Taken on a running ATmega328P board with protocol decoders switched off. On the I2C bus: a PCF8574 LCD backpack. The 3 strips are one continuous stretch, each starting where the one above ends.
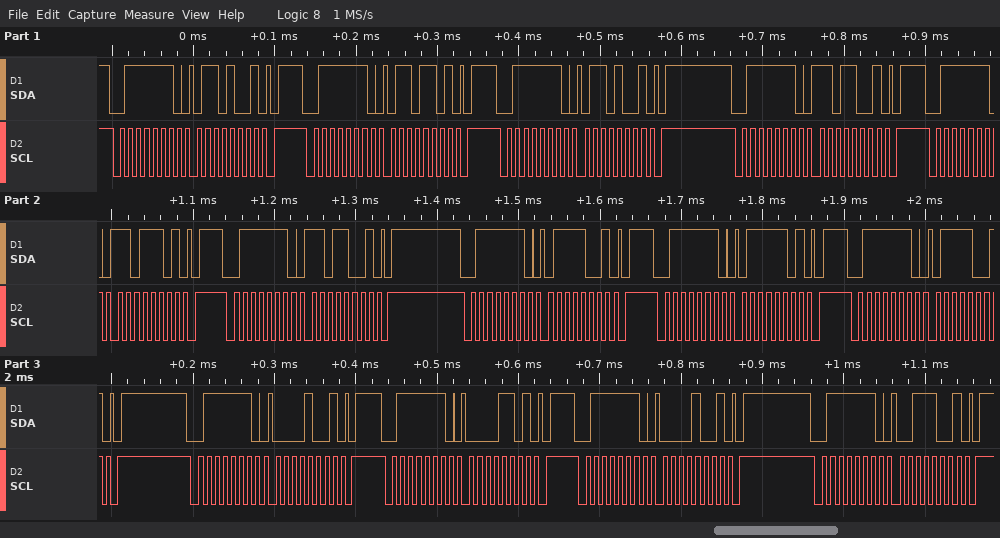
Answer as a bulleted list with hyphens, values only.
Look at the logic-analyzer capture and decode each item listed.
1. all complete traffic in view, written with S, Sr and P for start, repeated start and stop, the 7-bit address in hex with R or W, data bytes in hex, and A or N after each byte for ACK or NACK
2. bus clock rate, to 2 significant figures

- S 3FW A 69 A P S 3FW A 6D A P S 3FW A 69 A P S 3FW A D9 A P S 3FW A DD A P S 3FW A D9 A P S 3FW A 79 A P S 3FW A 7D A P S 3FW A 79 A P S 3FW A 09 A P S 3FW A 0D A P S 3FW A 09 A P S 3FW A 39 A P
- 100 kHz
